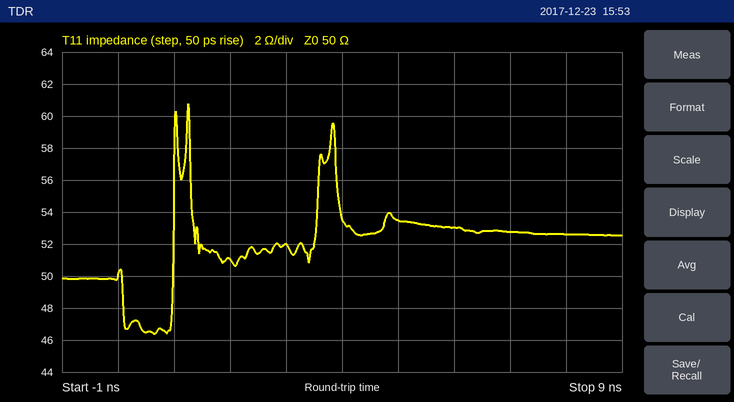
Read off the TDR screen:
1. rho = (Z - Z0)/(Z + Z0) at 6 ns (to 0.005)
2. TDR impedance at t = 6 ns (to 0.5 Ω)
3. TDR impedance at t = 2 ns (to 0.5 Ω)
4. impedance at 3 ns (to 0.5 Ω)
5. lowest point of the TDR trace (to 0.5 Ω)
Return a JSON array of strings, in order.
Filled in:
["+0.030", "53.0 Ω", "51.0 Ω", "52.0 Ω", "46.5 Ω"]
